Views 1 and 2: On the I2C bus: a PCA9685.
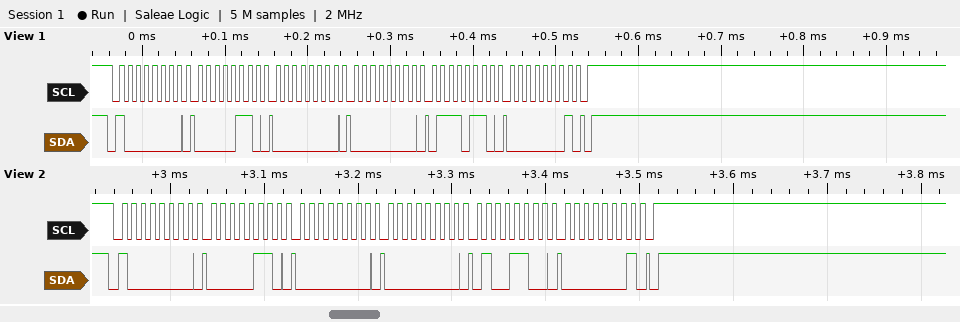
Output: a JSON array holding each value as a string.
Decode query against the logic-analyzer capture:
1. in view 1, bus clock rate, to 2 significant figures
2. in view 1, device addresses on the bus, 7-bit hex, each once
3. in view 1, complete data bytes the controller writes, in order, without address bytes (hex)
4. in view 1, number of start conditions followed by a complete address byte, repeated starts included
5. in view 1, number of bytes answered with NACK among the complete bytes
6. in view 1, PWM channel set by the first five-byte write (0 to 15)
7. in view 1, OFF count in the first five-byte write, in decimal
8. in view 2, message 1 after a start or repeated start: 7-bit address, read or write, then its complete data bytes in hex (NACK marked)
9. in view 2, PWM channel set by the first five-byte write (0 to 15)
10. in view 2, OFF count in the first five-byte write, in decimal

["100 kHz", "0x40", "06 00 00 76 01", "1", "0", "0", "374", "0x40 write: 06 00 00 4C 01", "0", "332"]
